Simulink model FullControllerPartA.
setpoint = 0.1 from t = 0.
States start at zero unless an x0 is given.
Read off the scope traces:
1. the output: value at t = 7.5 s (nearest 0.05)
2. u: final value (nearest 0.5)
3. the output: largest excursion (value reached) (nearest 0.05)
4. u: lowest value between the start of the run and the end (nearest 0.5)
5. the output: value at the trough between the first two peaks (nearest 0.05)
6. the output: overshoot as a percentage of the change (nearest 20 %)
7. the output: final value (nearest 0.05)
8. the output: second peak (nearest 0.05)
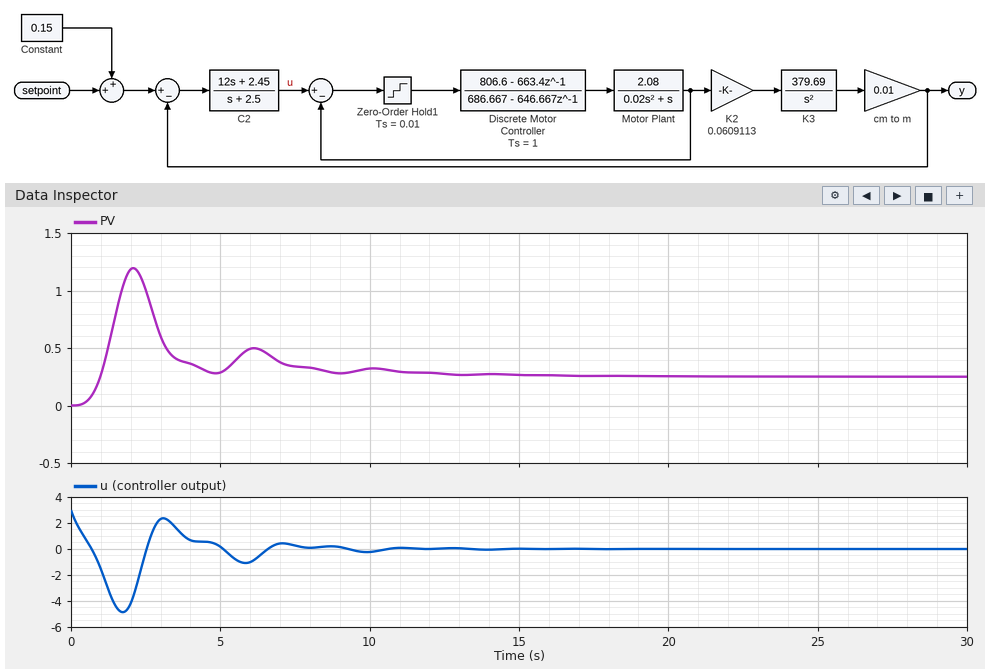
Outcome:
0.35
0.0
1.20
-5.0
0.30
380 %
0.25
0.50
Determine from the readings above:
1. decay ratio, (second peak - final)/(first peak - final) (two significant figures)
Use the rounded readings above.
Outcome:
0.26
